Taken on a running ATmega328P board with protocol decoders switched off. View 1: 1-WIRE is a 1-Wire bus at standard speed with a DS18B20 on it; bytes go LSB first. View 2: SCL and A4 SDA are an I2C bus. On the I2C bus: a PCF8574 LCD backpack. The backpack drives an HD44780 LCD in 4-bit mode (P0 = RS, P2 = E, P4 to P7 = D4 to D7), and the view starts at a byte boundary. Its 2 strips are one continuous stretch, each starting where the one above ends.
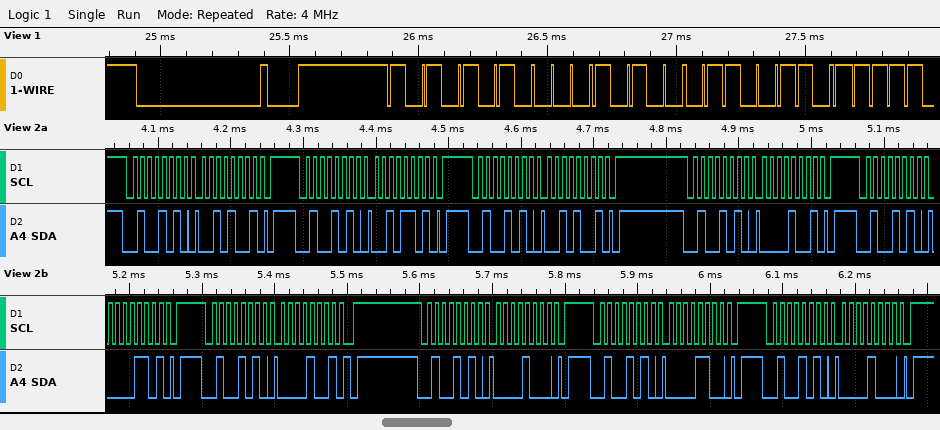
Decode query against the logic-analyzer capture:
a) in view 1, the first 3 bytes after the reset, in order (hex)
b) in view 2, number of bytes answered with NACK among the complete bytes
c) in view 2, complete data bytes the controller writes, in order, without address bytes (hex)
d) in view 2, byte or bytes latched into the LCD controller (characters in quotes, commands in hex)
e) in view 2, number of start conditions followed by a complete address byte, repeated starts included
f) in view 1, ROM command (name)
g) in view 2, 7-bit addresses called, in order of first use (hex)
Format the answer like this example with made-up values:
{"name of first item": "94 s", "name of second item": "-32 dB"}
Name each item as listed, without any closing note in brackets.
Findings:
{"in view 1, the first 3 bytes after the reset, in order": "55 28 66", "in view 2, number of bytes answered with NACK among the complete bytes": "0", "in view 2, complete data bytes the controller writes, in order, without address bytes": "29 2D 29 09 0D 09 08 0C 08", "in view 2, byte or bytes latched into the LCD controller": "' '", "in view 2, number of start conditions followed by a complete address byte, repeated starts included": "9", "in view 1, ROM command": "Match ROM", "in view 2, 7-bit addresses called, in order of first use": "0x25"}
